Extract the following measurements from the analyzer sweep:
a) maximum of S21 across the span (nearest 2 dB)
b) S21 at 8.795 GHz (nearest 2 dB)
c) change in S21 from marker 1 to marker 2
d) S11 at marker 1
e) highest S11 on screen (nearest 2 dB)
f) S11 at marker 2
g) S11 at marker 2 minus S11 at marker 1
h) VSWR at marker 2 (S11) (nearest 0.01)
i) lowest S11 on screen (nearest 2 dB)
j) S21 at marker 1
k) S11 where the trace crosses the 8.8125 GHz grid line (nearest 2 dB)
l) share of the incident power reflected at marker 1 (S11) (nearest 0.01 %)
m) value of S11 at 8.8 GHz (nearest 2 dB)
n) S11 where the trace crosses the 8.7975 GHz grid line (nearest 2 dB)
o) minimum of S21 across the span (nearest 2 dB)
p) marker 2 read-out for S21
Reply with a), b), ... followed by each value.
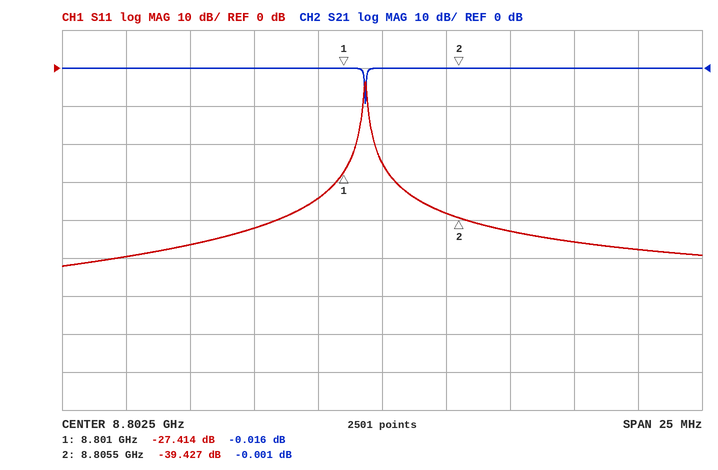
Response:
a) 0 dB
b) 0 dB
c) 0.015 dB
d) -27.414 dB
e) -4 dB
f) -39.427 dB
g) -12.013 dB
h) 1.02
i) -52 dB
j) -0.016 dB
k) -48 dB
l) 0.18 %
m) -34 dB
n) -42 dB
o) -10 dB
p) -0.001 dB
